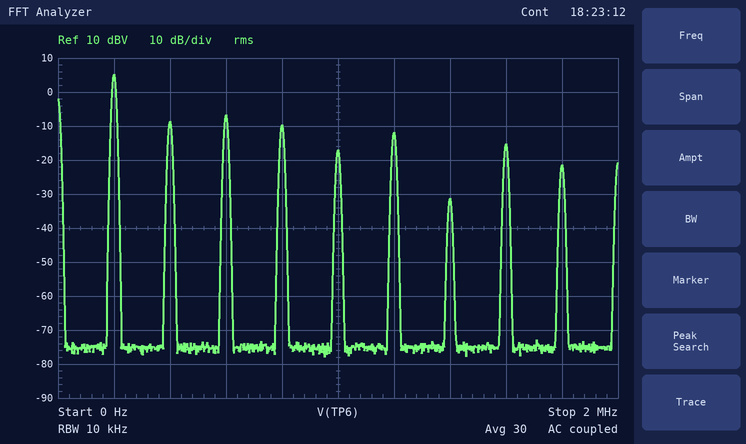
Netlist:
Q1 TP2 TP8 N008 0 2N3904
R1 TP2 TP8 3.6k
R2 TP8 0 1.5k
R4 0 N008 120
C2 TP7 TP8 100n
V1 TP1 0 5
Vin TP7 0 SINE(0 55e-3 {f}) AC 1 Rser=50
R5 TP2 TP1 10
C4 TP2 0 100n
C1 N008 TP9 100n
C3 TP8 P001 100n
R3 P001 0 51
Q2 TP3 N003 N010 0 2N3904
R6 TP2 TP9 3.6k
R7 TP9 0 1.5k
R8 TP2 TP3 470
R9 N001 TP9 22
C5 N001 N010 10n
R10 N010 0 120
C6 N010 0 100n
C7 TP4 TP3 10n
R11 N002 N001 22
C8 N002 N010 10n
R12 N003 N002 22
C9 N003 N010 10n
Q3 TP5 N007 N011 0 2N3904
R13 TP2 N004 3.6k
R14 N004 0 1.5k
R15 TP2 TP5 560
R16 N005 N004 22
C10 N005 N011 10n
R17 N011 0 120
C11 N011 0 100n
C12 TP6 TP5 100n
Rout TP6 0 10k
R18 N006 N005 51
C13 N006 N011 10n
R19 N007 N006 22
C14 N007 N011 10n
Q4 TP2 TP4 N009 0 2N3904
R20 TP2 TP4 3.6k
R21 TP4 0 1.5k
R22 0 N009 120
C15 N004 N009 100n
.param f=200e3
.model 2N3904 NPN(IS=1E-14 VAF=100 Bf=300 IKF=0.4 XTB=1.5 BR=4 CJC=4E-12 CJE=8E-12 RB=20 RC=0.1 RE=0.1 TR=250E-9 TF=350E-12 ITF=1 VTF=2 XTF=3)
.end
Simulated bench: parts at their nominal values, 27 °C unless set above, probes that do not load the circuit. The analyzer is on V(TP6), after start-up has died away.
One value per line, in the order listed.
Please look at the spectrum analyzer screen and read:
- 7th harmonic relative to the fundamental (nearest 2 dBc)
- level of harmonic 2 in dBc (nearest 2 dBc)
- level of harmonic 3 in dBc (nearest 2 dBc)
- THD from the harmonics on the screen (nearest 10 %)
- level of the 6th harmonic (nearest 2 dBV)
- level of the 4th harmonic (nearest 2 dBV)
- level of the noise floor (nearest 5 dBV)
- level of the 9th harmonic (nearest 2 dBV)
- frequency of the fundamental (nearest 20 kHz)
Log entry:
-36 dBc
-14 dBc
-12 dBc
40 %
-12 dBV
-10 dBV
-75 dBV
-22 dBV
200 kHz
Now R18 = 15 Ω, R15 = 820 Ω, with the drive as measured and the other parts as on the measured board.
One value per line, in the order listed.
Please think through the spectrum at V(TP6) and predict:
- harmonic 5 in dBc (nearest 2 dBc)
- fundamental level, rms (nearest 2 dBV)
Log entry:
-20 dBc
6 dBV
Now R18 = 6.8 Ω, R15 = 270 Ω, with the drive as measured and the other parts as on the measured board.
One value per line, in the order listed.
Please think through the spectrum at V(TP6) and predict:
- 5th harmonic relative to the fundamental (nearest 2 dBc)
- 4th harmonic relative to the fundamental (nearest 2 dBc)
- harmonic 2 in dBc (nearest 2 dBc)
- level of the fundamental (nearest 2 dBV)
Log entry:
-14 dBc
-12 dBc
-6 dBc
4 dBV
